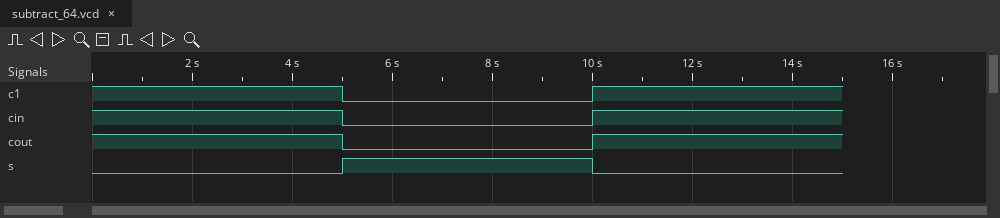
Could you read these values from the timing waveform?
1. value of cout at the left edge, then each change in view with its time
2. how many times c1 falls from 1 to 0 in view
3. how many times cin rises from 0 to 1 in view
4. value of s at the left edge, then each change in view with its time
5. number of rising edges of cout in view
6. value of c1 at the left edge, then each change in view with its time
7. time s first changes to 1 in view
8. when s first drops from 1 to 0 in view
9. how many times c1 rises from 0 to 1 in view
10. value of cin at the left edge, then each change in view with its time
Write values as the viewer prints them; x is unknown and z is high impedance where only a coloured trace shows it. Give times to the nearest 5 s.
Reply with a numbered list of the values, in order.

1. 1, 0 at 5 s, 1 at 10 s
2. 1
3. 1
4. 0, 1 at 5 s, 0 at 10 s
5. 1
6. 1, 0 at 5 s, 1 at 10 s
7. 5 s
8. 10 s
9. 1
10. 1, 0 at 5 s, 1 at 10 s
